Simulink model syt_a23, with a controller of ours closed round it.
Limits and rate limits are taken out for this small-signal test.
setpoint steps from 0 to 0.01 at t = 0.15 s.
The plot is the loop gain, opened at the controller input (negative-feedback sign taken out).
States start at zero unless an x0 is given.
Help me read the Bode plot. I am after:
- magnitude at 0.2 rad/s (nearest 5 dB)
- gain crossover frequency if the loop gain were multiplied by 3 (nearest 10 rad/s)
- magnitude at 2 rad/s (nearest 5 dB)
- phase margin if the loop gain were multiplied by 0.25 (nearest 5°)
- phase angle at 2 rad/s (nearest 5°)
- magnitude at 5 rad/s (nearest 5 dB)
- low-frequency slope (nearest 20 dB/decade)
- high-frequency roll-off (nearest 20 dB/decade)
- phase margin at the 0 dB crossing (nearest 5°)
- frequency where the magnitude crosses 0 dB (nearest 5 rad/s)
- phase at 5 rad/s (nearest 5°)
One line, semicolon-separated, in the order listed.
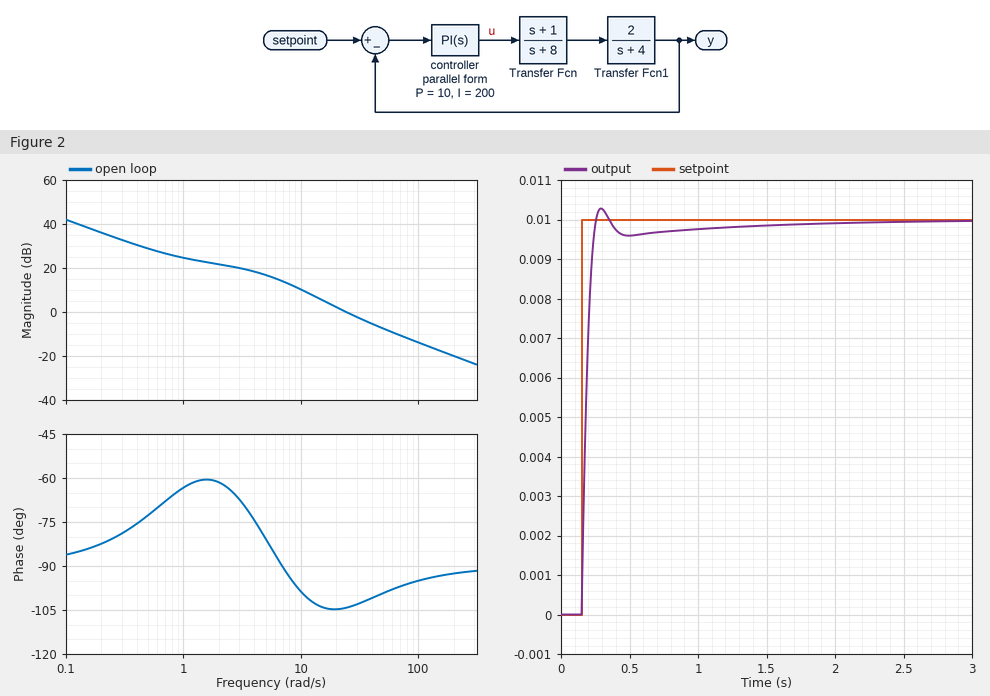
35 dB; 60 rad/s; 20 dB; 85°; -60°; 15 dB; -20 dB/decade; -20 dB/decade; 75°; 25 rad/s; -80°
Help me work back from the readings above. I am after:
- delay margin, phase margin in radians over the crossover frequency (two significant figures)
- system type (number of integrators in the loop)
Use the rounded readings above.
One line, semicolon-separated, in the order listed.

0.052 s; 1
